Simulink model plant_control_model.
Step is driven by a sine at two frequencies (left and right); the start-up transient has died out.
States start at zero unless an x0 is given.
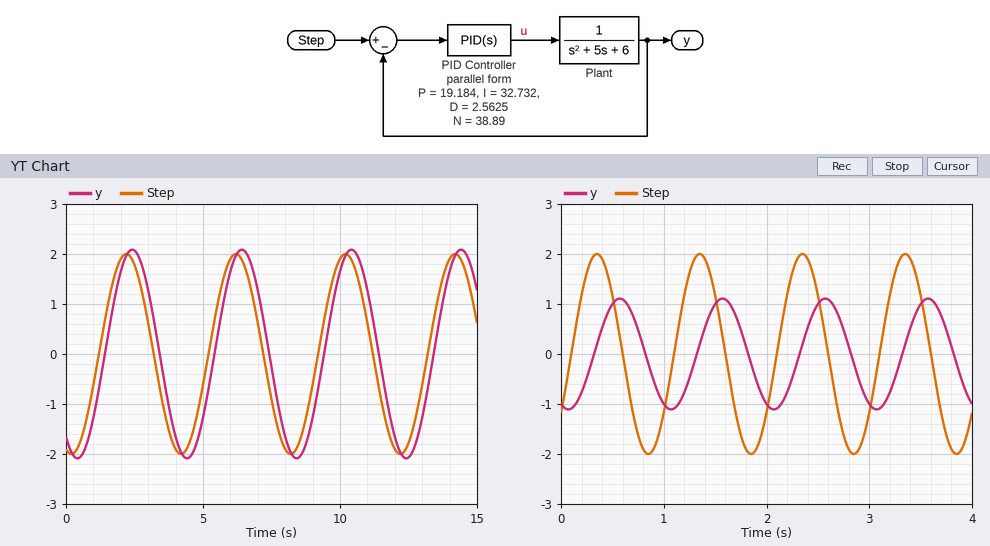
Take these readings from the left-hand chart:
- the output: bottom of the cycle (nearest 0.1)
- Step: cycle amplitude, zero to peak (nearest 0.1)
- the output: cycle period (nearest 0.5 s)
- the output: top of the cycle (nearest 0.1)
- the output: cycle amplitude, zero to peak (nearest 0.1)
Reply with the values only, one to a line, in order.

-2.1
2.0
4.0 s
2.1
2.1
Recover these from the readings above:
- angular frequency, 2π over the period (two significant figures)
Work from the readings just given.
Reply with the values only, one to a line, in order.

1.6 rad/s
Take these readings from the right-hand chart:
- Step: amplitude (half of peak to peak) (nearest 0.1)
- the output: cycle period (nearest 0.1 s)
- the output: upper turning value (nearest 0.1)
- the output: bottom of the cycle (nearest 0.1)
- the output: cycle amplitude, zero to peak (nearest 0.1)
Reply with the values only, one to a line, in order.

2.0
1.0 s
1.1
-1.1
1.1
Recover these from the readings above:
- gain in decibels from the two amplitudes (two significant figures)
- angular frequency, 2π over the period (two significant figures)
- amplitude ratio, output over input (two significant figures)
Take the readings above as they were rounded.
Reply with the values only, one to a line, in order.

-5.2 dB
6.3 rad/s
0.55
